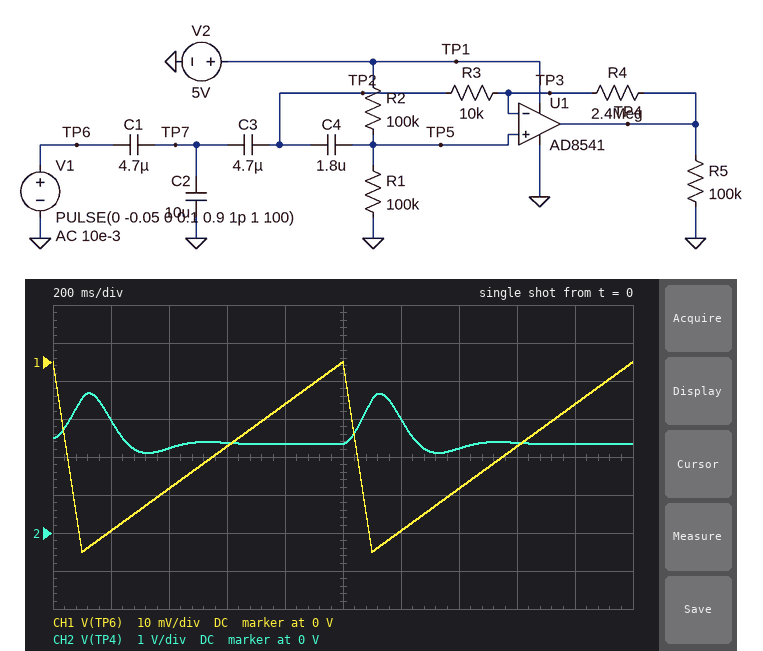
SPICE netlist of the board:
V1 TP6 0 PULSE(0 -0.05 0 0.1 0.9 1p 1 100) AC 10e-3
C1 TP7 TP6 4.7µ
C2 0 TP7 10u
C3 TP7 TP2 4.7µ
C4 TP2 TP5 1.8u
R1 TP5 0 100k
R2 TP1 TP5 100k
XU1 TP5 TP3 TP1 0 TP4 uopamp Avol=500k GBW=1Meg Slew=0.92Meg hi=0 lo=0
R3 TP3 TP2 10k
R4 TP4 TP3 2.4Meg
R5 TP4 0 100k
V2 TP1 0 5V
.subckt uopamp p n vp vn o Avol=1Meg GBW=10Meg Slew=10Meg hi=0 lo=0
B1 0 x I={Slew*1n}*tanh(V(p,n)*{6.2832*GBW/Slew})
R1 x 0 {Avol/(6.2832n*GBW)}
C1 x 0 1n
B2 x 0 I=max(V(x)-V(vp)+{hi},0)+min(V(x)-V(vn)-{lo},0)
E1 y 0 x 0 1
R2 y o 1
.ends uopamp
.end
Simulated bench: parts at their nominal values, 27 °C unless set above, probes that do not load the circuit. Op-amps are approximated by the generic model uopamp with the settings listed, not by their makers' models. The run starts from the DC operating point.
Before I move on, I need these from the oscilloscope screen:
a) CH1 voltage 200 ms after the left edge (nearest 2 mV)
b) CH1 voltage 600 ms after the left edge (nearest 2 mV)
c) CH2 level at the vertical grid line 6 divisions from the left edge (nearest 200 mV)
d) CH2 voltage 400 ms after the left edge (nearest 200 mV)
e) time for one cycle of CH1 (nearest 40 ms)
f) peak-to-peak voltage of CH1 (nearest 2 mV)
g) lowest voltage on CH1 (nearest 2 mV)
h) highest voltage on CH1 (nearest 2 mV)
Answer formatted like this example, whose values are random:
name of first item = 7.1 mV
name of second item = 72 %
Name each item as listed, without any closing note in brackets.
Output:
CH1 voltage 200 ms after the left edge = -44 mV
CH1 voltage 600 ms after the left edge = -22 mV
CH2 level at the vertical grid line 6 divisions from the left edge = 3.0 V
CH2 voltage 400 ms after the left edge = 2.2 V
time for one cycle of CH1 = 1.00 s
peak-to-peak voltage of CH1 = 50 mV
lowest voltage on CH1 = -50 mV
highest voltage on CH1 = 0 V
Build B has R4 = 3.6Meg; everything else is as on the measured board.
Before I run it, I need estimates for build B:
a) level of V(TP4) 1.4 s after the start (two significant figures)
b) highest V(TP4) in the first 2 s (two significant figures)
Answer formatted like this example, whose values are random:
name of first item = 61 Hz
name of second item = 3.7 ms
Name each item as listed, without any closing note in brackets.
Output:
level of V(TP4) 1.4 s after the start = 2.1 V
highest V(TP4) in the first 2 s = 4.3 V
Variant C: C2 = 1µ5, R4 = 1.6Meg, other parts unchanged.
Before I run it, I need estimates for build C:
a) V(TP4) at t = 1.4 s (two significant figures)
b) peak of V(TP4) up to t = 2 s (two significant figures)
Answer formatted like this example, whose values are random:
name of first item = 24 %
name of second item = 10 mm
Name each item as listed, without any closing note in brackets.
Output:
V(TP4) at t = 1.4 s = 2.3 V
peak of V(TP4) up to t = 2 s = 4.1 V
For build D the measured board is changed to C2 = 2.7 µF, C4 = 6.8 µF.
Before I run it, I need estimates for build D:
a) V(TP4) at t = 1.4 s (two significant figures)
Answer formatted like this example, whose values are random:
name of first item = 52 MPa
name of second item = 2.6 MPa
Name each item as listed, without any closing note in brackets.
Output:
V(TP4) at t = 1.4 s = 2.3 V
